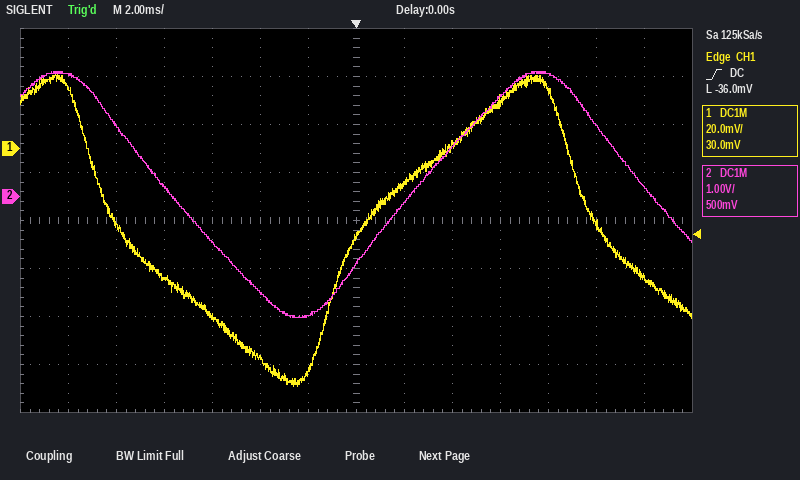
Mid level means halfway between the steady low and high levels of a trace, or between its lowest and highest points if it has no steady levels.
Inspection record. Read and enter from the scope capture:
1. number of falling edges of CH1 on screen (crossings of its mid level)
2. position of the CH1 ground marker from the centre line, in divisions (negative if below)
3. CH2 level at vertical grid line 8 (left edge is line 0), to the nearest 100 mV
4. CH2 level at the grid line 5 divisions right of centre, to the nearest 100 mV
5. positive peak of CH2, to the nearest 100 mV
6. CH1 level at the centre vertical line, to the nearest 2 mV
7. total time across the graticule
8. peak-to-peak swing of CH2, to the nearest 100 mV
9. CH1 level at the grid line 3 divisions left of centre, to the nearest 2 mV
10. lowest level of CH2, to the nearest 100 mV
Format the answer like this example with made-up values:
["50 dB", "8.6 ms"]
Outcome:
["2", "+1.5 div", "-100 mV", "1.5 V", "2.6 V", "-36 mV", "28 ms", "5.1 V", "-70 mV", "-2.5 V"]
